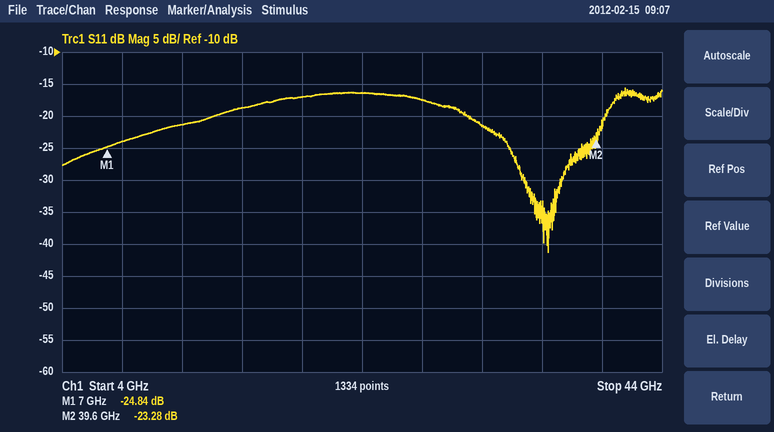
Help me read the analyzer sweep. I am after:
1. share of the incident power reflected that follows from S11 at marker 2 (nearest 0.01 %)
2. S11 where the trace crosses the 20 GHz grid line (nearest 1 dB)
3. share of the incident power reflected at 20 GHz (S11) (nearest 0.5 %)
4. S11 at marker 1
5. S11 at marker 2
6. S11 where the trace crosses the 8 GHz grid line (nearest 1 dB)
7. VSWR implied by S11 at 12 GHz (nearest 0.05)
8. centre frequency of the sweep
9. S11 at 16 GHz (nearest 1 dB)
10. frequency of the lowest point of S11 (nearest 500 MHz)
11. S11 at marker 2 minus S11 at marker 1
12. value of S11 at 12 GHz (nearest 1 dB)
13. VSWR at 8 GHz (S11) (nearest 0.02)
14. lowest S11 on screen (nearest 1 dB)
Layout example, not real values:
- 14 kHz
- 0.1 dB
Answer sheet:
- 0.47 %
- -17 dB
- 2.0 %
- -24.84 dB
- -23.28 dB
- -24 dB
- 1.20
- 24 GHz
- -19 dB
- 36.5 GHz
- 1.56 dB
- -21 dB
- 1.14
- -41 dB
